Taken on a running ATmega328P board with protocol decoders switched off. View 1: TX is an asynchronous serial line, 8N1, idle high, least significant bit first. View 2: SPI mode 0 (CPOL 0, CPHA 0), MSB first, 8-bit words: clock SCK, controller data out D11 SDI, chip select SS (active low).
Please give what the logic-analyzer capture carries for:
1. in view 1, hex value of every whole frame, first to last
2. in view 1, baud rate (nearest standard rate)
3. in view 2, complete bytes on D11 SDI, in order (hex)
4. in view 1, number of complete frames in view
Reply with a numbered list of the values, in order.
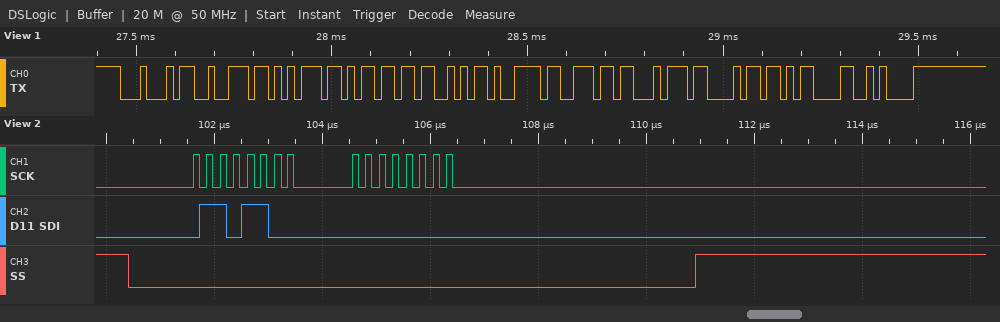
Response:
1. 44 72 75 6D 53 79 6E 74 68 0D 0A
2. 57600 baud
3. 0x6C 0x00
4. 11
